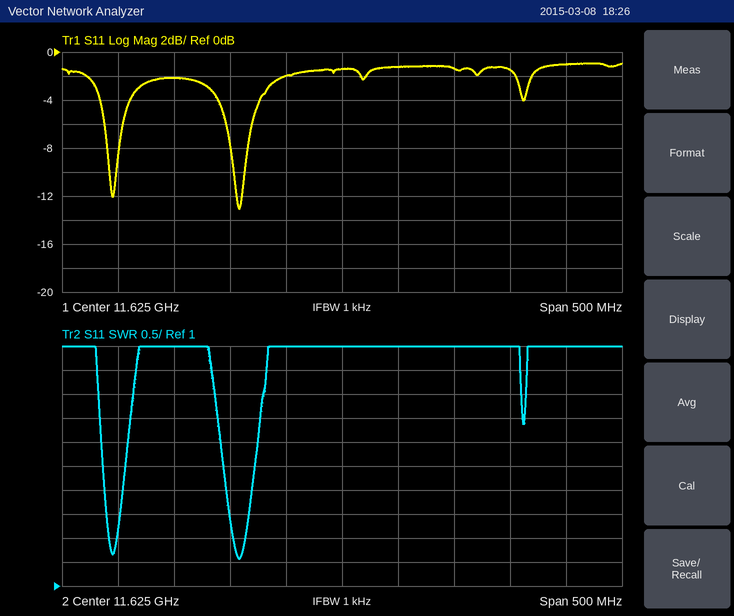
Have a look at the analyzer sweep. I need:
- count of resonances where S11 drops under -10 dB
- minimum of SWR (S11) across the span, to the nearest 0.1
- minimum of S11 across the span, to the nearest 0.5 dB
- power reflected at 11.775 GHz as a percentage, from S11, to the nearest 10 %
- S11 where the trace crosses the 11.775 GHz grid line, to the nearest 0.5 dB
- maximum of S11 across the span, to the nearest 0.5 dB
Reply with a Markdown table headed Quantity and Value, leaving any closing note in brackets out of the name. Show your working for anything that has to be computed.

| Quantity | Value |
|---|---|
| count of resonances where S11 drops under -10 dB | 2 |
| minimum of SWR (S11) across the span, to the nearest 0.1 | 1.6 |
| minimum of S11 across the span, to the nearest 0.5 dB | -13.0 dB |
| power reflected at 11.775 GHz as a percentage, from S11, to the nearest 10 % | 10^(-1.5/10) ≈ 70.8 %, so 70 % to the nearest 10 % |
| S11 where the trace crosses the 11.775 GHz grid line, to the nearest 0.5 dB | -1.5 dB |
| maximum of S11 across the span, to the nearest 0.5 dB | -1.0 dB |
